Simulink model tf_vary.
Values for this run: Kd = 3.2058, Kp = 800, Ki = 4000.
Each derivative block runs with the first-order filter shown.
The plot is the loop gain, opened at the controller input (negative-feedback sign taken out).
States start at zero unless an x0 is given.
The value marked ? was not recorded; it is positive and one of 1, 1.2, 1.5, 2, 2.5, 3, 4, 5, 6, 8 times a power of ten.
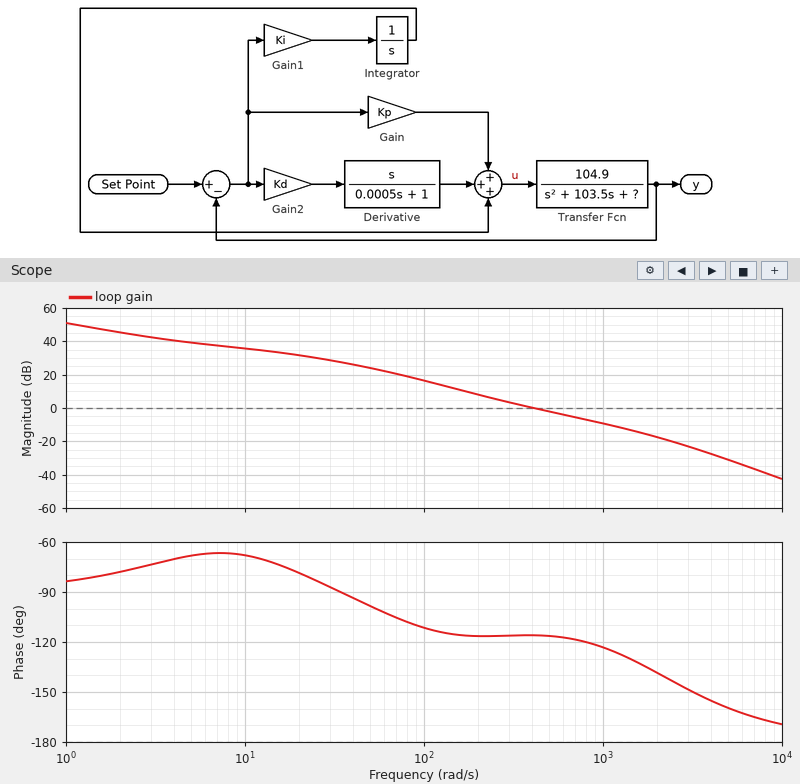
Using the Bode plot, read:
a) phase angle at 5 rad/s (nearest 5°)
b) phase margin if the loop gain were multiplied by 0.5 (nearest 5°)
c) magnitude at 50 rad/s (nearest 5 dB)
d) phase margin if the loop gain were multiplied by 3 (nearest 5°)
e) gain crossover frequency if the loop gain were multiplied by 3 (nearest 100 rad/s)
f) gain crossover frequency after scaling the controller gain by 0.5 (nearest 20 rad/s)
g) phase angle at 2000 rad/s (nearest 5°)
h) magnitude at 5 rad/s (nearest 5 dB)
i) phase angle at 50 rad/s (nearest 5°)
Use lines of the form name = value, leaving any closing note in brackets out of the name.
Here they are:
phase angle at 5 rad/s = -70°
phase margin if the loop gain were multiplied by 0.5 = 65°
magnitude at 50 rad/s = 25 dB
phase margin if the loop gain were multiplied by 3 = 55°
gain crossover frequency if the loop gain were multiplied by 3 = 1000 rad/s
gain crossover frequency after scaling the controller gain by 0.5 = 240 rad/s
phase angle at 2000 rad/s = -140°
magnitude at 5 rad/s = 40 dB
phase angle at 50 rad/s = -100°
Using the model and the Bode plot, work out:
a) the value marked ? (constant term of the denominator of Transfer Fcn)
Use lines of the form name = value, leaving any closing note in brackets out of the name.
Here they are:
the value marked ? = 1200
